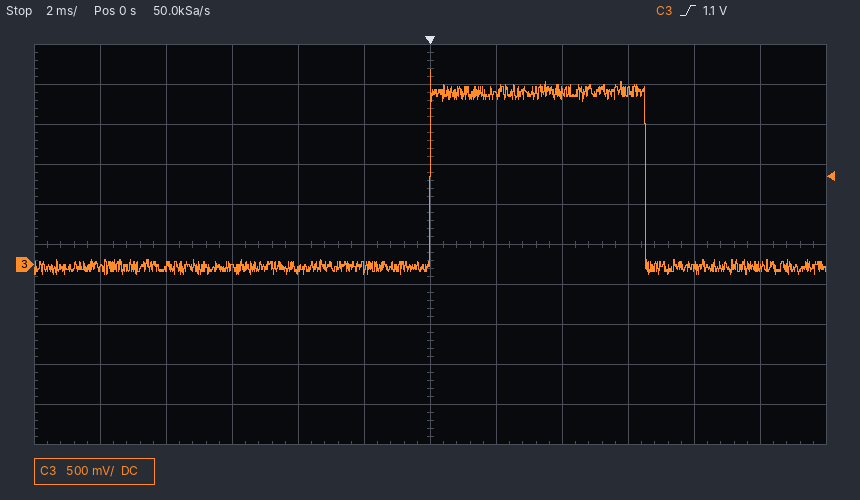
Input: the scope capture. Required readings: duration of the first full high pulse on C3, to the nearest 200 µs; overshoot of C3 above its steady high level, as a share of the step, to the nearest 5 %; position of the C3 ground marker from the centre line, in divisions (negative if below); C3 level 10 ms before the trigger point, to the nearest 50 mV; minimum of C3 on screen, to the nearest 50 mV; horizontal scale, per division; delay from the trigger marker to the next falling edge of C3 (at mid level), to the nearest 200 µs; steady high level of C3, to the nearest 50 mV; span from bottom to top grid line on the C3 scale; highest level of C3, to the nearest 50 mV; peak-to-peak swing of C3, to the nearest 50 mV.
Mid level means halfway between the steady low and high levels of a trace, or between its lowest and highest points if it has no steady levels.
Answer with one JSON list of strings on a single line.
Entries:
["6.6 ms", "15 %", "-0.5 div", "-50 mV", "-100 mV", "2 ms", "6.6 ms", "2.15 V", "5 V", "2.45 V", "2.55 V"]
